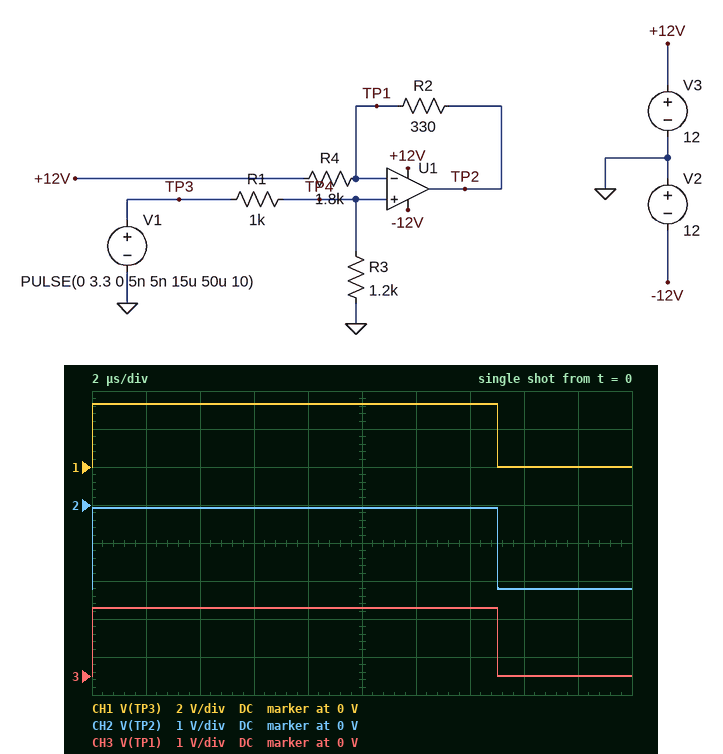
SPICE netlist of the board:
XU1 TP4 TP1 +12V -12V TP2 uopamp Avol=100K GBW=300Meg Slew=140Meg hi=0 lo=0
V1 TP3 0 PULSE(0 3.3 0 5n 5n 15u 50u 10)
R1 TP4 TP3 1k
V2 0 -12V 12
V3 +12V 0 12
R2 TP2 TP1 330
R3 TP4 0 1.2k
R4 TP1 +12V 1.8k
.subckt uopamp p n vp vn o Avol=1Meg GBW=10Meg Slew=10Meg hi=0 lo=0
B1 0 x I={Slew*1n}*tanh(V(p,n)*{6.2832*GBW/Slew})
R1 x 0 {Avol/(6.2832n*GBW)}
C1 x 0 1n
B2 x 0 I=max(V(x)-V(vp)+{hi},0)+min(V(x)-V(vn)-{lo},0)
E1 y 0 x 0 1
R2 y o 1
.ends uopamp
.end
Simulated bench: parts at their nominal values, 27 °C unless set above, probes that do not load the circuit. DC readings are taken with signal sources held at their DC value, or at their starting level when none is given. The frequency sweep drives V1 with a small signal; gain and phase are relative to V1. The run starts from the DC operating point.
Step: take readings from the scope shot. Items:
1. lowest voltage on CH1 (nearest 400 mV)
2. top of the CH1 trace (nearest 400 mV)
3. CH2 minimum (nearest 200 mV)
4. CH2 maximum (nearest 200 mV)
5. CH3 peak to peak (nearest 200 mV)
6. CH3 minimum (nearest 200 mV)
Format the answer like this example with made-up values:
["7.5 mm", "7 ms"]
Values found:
["0 V", "3.2 V", "-2.2 V", "0 V", "1.8 V", "0 V"]
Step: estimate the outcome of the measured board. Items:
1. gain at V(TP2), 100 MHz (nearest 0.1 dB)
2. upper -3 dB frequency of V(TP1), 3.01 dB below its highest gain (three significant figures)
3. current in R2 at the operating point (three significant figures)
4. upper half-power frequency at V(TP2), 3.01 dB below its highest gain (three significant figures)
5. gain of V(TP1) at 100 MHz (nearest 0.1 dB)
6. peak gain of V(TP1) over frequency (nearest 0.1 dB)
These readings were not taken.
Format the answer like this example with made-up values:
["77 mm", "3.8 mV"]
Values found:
["-4.4 dB", "253 MHz", "6.67 mA", "253 MHz", "-5.9 dB", "-5.3 dB"]
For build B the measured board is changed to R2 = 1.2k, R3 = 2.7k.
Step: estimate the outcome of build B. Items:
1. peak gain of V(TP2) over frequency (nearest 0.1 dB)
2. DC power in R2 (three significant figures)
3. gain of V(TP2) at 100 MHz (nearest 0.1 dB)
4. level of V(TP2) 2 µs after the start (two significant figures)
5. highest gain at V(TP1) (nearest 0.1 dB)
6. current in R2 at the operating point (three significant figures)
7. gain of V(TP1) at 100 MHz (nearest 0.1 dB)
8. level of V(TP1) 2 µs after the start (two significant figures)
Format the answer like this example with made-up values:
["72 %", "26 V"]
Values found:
["1.7 dB", "53.3 mW", "0.5 dB", "-4.0 V", "-2.7 dB", "6.67 mA", "-3.9 dB", "2.4 V"]
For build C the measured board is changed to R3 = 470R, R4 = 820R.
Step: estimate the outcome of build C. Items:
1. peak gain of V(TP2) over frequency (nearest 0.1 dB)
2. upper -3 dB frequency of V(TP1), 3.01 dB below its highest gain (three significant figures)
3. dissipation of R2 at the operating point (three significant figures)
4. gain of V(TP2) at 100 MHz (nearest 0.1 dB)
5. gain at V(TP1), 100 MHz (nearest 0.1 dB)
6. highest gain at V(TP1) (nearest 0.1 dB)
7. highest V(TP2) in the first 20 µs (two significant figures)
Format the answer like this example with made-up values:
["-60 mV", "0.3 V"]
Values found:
["-7.0 dB", "214 MHz", "70.7 mW", "-7.8 dB", "-10.8 dB", "-9.9 dB", "-3.3 V"]
